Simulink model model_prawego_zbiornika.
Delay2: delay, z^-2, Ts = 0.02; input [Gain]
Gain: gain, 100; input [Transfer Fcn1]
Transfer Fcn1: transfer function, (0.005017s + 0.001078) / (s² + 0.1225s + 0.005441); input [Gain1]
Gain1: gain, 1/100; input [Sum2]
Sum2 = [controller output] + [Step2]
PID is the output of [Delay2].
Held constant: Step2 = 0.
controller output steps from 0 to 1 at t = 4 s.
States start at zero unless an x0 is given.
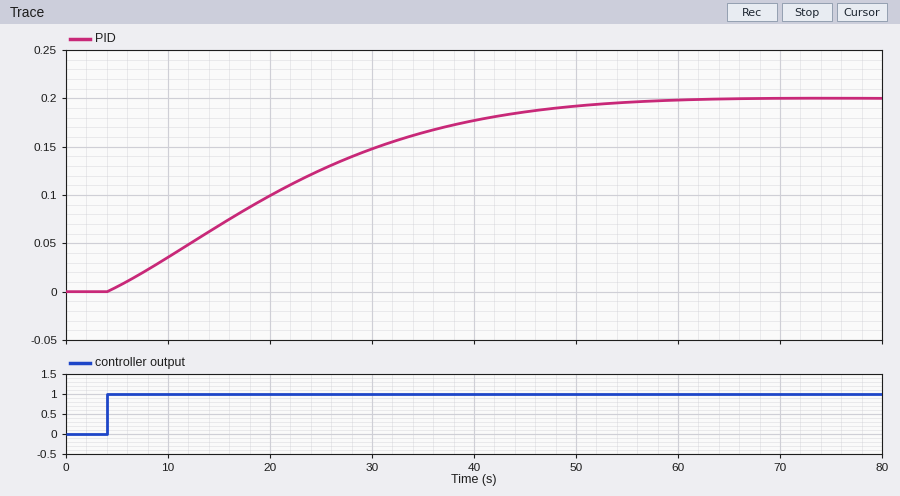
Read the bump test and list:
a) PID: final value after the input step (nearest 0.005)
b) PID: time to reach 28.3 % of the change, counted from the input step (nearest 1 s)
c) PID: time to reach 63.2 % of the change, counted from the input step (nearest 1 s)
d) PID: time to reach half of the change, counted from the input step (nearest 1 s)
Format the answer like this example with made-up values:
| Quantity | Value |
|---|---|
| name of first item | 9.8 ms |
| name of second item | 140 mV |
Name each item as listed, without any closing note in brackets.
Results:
| Quantity | Value |
|---|---|
| PID: final value after the input step | 0.200 |
| PID: time to reach 28.3 % of the change, counted from the input step | 9 s |
| PID: time to reach 63.2 % of the change, counted from the input step | 21 s |
| PID: time to reach half of the change, counted from the input step | 16 s |
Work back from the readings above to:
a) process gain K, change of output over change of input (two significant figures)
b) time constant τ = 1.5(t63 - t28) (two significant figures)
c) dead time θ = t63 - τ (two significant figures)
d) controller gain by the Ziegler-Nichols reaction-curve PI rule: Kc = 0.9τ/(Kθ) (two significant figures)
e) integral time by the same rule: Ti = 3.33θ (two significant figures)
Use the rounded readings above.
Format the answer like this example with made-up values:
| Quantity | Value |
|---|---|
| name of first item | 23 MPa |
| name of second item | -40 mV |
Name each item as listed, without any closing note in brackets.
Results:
| Quantity | Value |
|---|---|
| process gain K, change of output over change of input | 0.20 |
| time constant τ = 1.5(t63 - t28) | 18 s |
| dead time θ = t63 - τ | 3.0 s |
| controller gain by the Ziegler-Nichols reaction-curve PI rule: Kc = 0.9τ/(Kθ) | 27 |
| integral time by the same rule: Ti = 3.33θ | 10.0 s |
